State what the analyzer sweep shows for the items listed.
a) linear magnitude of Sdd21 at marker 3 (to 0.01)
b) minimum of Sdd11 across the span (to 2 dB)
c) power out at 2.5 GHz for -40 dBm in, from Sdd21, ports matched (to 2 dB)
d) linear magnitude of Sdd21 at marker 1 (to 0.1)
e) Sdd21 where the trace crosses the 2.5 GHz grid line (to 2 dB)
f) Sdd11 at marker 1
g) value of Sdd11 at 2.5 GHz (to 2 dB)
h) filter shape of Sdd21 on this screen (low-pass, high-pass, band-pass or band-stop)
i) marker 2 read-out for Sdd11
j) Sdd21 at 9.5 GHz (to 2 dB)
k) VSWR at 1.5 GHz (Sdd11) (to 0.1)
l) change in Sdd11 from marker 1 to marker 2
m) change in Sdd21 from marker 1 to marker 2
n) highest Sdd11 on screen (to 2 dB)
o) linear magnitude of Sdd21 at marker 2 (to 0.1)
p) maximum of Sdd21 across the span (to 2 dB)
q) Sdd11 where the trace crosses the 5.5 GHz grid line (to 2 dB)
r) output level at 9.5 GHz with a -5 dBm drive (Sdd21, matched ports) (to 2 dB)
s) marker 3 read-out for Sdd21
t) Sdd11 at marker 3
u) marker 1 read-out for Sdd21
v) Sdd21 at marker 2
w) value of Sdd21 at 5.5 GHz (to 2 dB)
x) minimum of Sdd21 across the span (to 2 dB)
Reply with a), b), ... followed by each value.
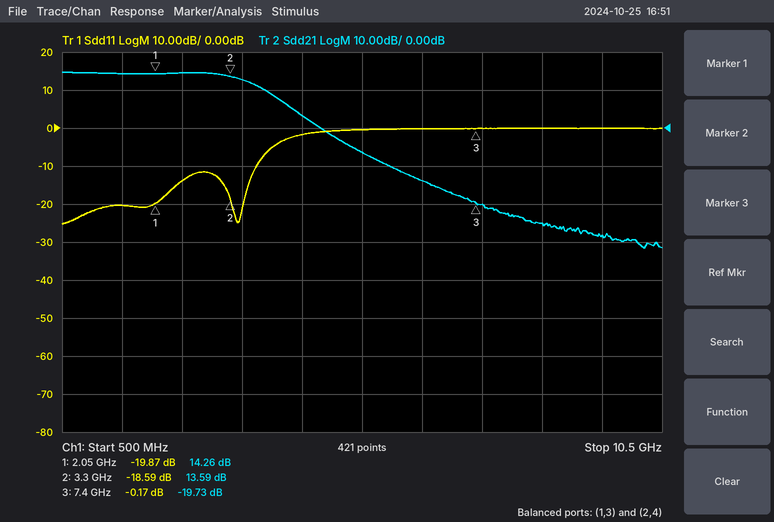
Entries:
a) 0.10
b) -26 dB
c) -26 dBm
d) 5.2
e) 14 dB
f) -19.87 dB
g) -14 dB
h) low-pass
i) -18.59 dB
j) -28 dB
k) 1.2
l) 1.28 dB
m) -0.67 dB
n) 0 dB
o) 4.8
p) 14 dB
q) 0 dB
r) -34 dBm
s) -19.73 dB
t) -0.17 dB
u) 14.26 dB
v) 13.59 dB
w) -6 dB
x) -32 dB
